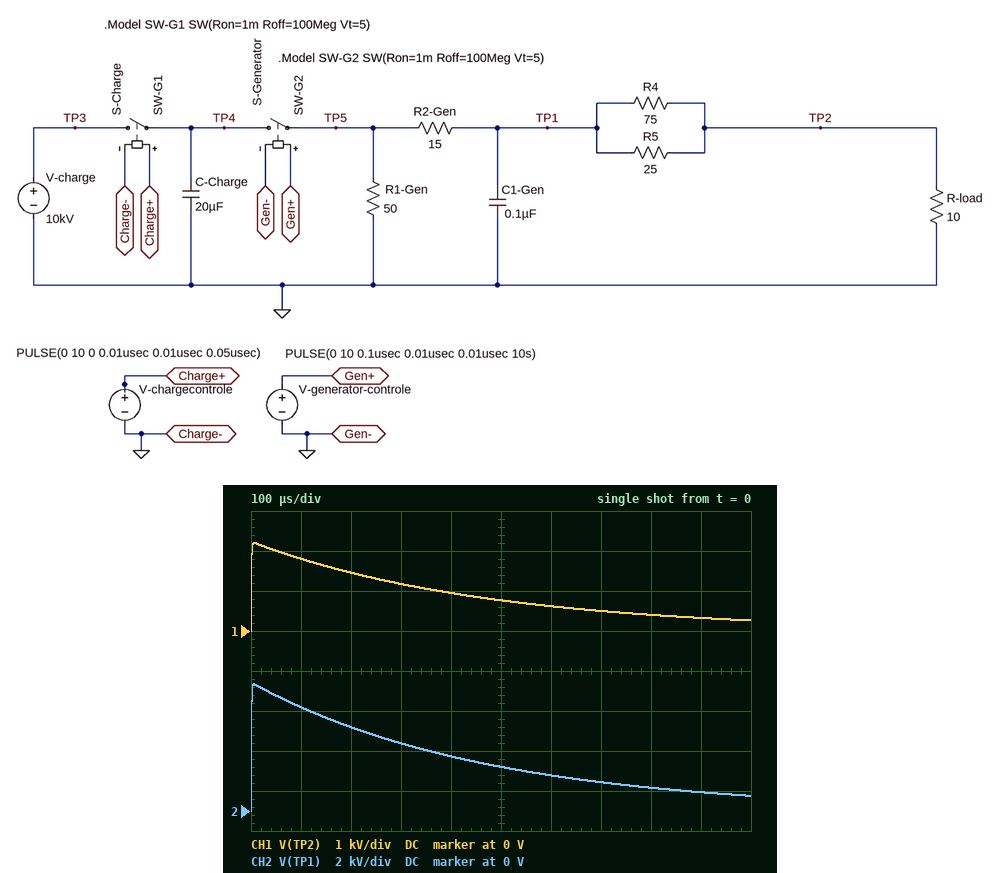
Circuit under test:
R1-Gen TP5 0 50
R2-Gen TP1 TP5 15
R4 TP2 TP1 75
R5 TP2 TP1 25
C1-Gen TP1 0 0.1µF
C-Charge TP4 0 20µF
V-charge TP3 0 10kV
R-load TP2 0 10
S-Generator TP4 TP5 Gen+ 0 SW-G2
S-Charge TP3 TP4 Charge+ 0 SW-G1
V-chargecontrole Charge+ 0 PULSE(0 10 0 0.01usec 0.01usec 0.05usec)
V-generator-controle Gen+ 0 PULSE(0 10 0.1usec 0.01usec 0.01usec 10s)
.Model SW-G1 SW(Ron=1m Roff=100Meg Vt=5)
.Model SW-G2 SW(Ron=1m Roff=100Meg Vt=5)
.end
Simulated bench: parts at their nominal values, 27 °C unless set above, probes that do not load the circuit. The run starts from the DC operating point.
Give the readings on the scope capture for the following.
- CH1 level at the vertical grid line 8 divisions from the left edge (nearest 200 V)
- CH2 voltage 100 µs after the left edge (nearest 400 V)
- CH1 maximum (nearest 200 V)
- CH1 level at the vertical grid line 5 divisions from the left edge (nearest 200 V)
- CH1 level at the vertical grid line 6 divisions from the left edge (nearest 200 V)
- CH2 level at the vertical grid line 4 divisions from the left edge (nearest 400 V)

400 V
5.2 kV
2.2 kV
800 V
600 V
2.8 kV
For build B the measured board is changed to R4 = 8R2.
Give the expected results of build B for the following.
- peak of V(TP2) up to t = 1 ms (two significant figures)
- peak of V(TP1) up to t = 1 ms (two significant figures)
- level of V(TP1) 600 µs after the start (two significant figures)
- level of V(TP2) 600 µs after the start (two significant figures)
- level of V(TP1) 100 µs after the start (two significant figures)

3.1 kV
5.0 kV
1.1 kV
660 V
3.9 kV
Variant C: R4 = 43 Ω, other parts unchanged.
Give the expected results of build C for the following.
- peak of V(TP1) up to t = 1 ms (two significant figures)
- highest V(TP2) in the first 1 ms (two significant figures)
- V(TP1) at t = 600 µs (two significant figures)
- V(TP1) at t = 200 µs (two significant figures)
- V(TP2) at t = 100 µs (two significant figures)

6.1 kV
2.4 kV
1.6 kV
4.0 kV
1.9 kV
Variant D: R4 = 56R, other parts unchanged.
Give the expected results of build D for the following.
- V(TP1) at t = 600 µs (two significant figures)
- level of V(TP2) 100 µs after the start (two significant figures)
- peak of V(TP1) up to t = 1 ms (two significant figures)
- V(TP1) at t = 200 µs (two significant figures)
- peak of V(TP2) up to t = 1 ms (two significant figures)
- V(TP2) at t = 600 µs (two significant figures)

1.7 kV
1.9 kV
6.2 kV
4.1 kV
2.3 kV
630 V
